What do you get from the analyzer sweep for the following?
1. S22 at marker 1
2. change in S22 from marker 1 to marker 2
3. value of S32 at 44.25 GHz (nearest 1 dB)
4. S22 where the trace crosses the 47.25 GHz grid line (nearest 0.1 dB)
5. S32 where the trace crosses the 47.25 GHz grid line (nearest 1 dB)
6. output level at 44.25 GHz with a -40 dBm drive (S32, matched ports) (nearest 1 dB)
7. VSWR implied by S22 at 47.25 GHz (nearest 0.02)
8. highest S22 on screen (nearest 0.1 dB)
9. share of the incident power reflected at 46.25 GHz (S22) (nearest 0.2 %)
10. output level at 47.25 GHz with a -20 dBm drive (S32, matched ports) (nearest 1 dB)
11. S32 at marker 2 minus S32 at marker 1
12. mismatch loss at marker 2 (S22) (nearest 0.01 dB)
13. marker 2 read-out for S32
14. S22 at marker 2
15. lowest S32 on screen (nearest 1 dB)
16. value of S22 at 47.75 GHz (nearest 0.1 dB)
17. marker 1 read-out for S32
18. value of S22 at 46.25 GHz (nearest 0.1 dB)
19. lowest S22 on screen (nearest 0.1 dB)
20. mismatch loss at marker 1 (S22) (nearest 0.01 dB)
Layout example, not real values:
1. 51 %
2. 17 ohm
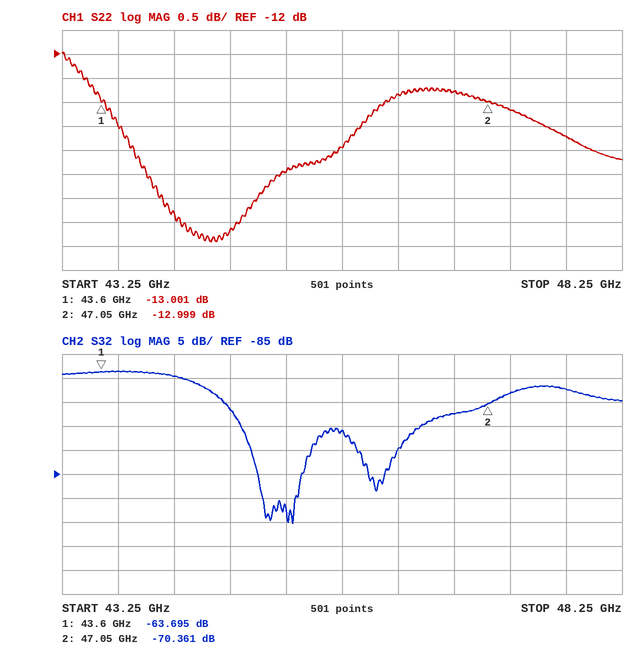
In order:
1. -13.001 dB
2. 0.002 dB
3. -65 dB
4. -13.2 dB
5. -68 dB
6. -105 dBm
7. 1.56
8. -12.0 dB
9. 5.2 %
10. -88 dBm
11. -6.666 dB
12. 0.22 dB
13. -70.361 dB
14. -12.999 dB
15. -95 dB
16. -13.7 dB
17. -63.695 dB
18. -12.8 dB
19. -15.9 dB
20. 0.22 dB
